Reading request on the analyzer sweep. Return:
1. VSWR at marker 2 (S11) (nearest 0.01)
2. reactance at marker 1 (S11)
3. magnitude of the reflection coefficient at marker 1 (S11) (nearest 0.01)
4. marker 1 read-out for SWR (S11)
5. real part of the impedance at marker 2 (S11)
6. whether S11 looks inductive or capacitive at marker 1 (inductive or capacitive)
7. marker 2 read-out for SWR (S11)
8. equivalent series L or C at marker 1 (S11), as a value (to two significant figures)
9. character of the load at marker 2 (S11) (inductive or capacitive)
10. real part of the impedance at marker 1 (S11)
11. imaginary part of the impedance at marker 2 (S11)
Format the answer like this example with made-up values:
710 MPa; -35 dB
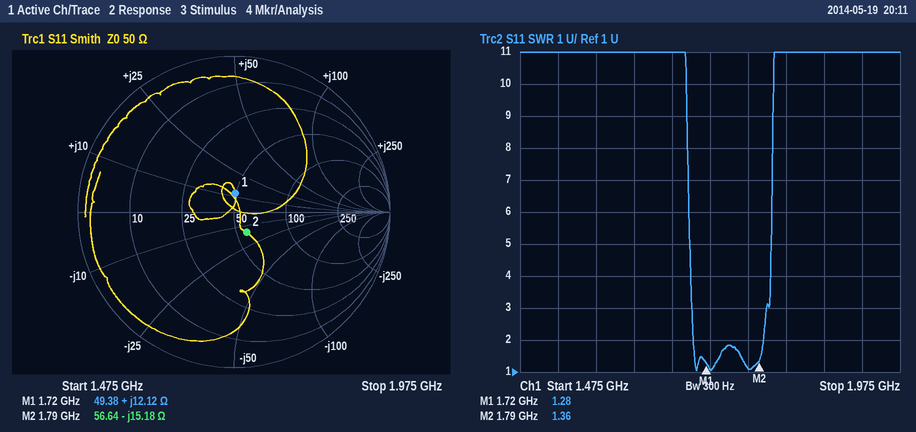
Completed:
1.36; +12.12 Ω; 0.12; 1.28; 56.64 Ω; inductive; 1.36; 1.1 nH; capacitive; 49.38 Ω; -15.18 Ω
